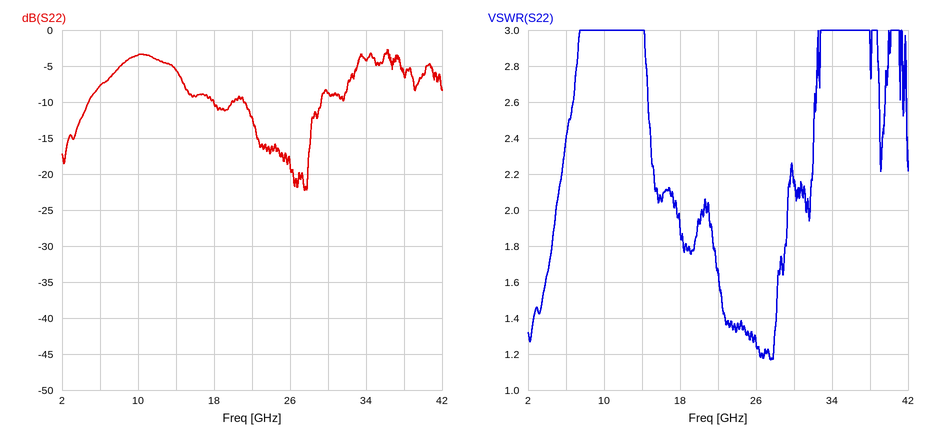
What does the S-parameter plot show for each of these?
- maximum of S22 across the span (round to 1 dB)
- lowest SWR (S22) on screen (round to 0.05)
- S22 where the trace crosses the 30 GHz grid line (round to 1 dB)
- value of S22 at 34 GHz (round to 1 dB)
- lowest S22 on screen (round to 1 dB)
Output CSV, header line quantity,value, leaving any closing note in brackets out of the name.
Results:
quantity,value
maximum of S22 across the span,-3 dB
lowest SWR (S22) on screen,1.15
S22 where the trace crosses the 30 GHz grid line,-9 dB
value of S22 at 34 GHz,-4 dB
lowest S22 on screen,-22 dB
